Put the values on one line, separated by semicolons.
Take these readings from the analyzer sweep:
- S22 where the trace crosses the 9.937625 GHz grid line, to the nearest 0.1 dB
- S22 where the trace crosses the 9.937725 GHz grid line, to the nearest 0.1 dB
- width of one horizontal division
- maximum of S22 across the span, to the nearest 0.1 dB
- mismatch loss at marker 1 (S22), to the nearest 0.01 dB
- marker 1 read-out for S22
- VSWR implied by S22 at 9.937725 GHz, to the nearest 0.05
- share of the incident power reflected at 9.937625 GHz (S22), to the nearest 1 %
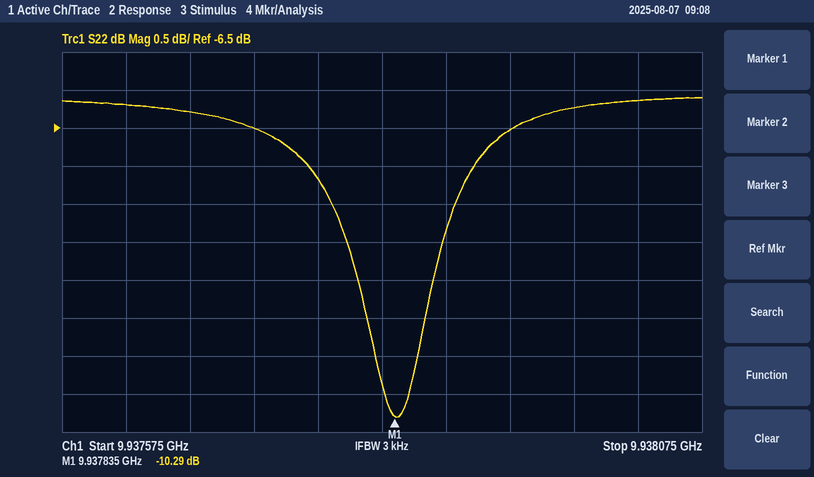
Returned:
-6.2 dB; -6.5 dB; 50 kHz; -6.1 dB; 0.43 dB; -10.29 dB; 2.80; 24 %
